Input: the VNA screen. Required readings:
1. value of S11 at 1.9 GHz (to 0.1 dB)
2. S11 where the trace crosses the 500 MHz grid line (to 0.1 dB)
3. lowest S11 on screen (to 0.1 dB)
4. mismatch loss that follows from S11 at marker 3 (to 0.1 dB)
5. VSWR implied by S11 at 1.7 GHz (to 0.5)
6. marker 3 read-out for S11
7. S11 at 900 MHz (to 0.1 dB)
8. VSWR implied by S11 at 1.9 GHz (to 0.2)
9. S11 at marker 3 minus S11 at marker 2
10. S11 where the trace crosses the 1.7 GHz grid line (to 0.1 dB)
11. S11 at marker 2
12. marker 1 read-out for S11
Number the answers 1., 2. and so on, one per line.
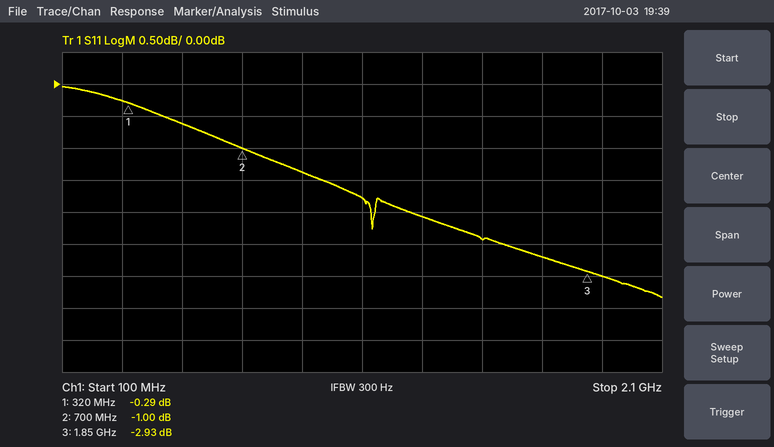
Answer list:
1. -3.0 dB
2. -0.6 dB
3. -3.3 dB
4. 3.1 dB
5. 6.5
6. -2.93 dB
7. -1.4 dB
8. 5.8
9. -1.93 dB
10. -2.7 dB
11. -1.00 dB
12. -0.29 dB
